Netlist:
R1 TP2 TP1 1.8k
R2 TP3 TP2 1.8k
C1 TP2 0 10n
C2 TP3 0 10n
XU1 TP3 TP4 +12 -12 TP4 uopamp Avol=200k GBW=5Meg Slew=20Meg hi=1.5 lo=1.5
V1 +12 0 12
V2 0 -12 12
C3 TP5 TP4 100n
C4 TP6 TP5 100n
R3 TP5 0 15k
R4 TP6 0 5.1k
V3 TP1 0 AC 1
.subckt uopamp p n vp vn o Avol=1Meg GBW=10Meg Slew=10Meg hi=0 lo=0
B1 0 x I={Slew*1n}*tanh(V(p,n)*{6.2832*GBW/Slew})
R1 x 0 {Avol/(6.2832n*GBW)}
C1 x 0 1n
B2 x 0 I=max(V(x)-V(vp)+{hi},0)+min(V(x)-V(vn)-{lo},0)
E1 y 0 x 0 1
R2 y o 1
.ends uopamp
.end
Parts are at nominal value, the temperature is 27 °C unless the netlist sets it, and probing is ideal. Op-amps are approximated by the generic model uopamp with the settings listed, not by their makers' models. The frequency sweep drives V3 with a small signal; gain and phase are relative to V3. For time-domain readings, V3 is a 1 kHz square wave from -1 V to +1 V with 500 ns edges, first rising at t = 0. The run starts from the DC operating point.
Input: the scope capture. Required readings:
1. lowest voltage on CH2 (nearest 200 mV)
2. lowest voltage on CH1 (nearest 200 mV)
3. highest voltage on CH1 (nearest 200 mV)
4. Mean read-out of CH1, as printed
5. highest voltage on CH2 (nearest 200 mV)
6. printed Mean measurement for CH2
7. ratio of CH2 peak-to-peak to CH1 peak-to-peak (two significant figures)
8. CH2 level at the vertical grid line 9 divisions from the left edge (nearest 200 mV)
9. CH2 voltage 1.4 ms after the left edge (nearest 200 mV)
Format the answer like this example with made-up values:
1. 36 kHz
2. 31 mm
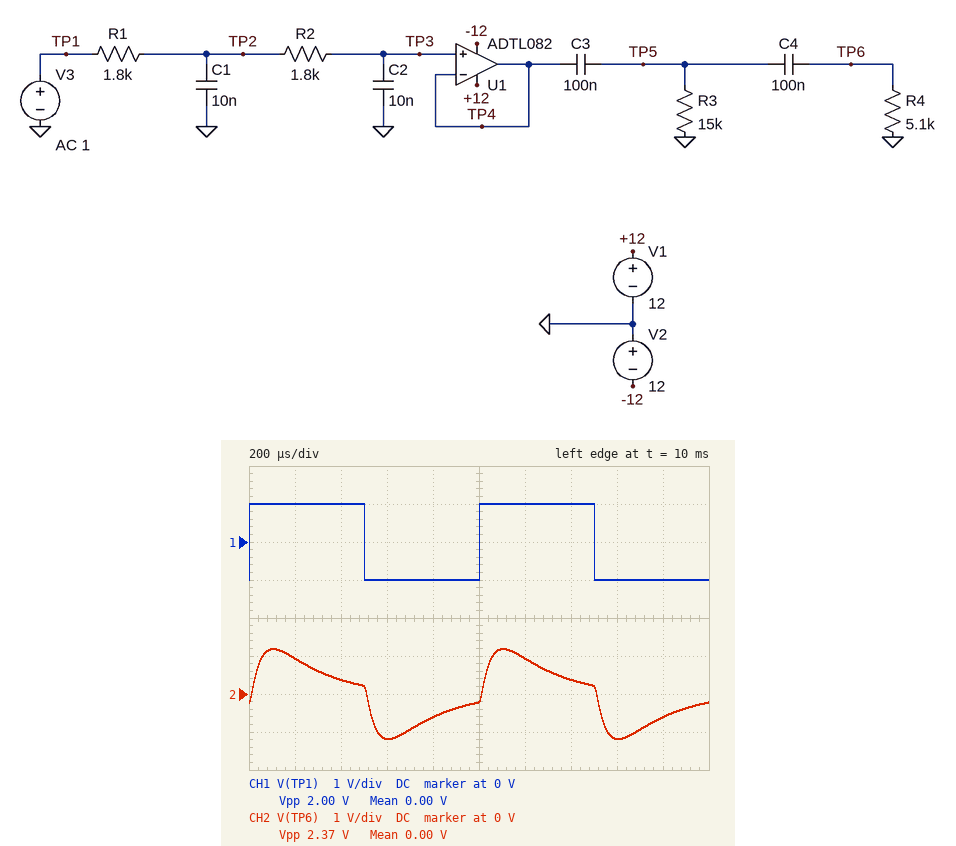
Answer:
1. -1.2 V
2. -1.0 V
3. 1.0 V
4. 0.00 V
5. 1.2 V
6. 0.00 V
7. 1.2
8. -600 mV
9. 400 mV
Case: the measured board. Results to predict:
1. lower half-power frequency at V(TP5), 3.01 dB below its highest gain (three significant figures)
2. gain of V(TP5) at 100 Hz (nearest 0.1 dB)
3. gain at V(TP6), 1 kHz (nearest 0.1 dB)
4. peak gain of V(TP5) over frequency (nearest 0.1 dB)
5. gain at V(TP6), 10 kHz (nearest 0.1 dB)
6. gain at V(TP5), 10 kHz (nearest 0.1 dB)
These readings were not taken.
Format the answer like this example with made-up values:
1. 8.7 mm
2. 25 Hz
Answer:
1. 346 Hz
2. -7.4 dB
3. -2.0 dB
4. -1.4 dB
5. -10.7 dB
6. -10.7 dB
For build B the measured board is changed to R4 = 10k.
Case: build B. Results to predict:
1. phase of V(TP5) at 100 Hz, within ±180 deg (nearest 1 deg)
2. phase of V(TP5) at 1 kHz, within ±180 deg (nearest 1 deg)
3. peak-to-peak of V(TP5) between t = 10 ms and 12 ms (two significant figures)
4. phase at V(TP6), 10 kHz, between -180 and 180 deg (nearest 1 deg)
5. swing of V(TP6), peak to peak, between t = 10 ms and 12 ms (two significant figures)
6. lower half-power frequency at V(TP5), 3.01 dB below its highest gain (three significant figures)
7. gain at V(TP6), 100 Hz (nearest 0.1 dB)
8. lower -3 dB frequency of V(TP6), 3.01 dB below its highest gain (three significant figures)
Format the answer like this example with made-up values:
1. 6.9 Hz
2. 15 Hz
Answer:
1. 39 deg
2. -5 deg
3. 2.1 V
4. -92 deg
5. 2.3 V
6. 251 Hz
7. -12.7 dB
8. 319 Hz
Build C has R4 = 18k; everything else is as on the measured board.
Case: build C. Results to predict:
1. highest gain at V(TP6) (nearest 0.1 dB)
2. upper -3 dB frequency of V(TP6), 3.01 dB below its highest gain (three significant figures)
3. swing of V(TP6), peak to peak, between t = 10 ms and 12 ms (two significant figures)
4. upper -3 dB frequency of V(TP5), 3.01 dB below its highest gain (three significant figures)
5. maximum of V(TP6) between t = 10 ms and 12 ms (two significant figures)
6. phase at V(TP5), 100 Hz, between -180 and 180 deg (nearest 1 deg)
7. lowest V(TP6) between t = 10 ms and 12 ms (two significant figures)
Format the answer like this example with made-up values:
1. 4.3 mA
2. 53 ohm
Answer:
1. -0.6 dB
2. 3.76 kHz
3. 2.2 V
4. 3.73 kHz
5. 1.1 V
6. 45 deg
7. -1.1 V
